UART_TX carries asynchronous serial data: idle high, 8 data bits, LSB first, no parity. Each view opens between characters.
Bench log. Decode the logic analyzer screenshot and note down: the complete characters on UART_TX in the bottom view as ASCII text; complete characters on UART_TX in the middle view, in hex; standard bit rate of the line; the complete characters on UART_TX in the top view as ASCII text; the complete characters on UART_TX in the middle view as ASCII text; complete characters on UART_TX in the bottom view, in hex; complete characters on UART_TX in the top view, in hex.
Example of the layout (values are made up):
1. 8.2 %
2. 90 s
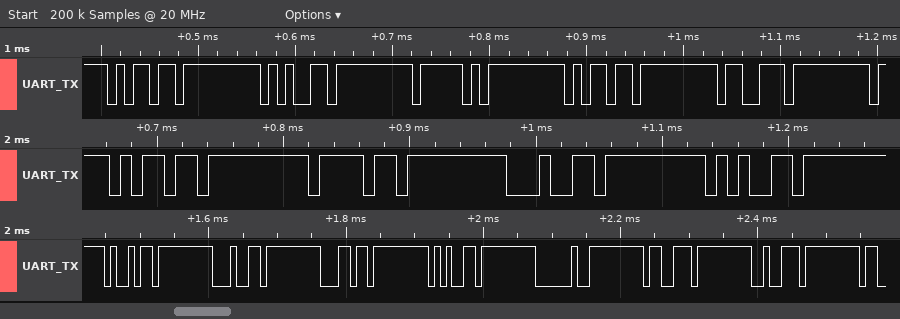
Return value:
1. "idle sr"
2. 6D, 6F, 64, 65
3. 115200 baud
4. "me_ms"
5. "mode"
6. 69, 64, 6C, 65, 20, 73, 72
7. 6D, 65, 5F, 6D, 73
